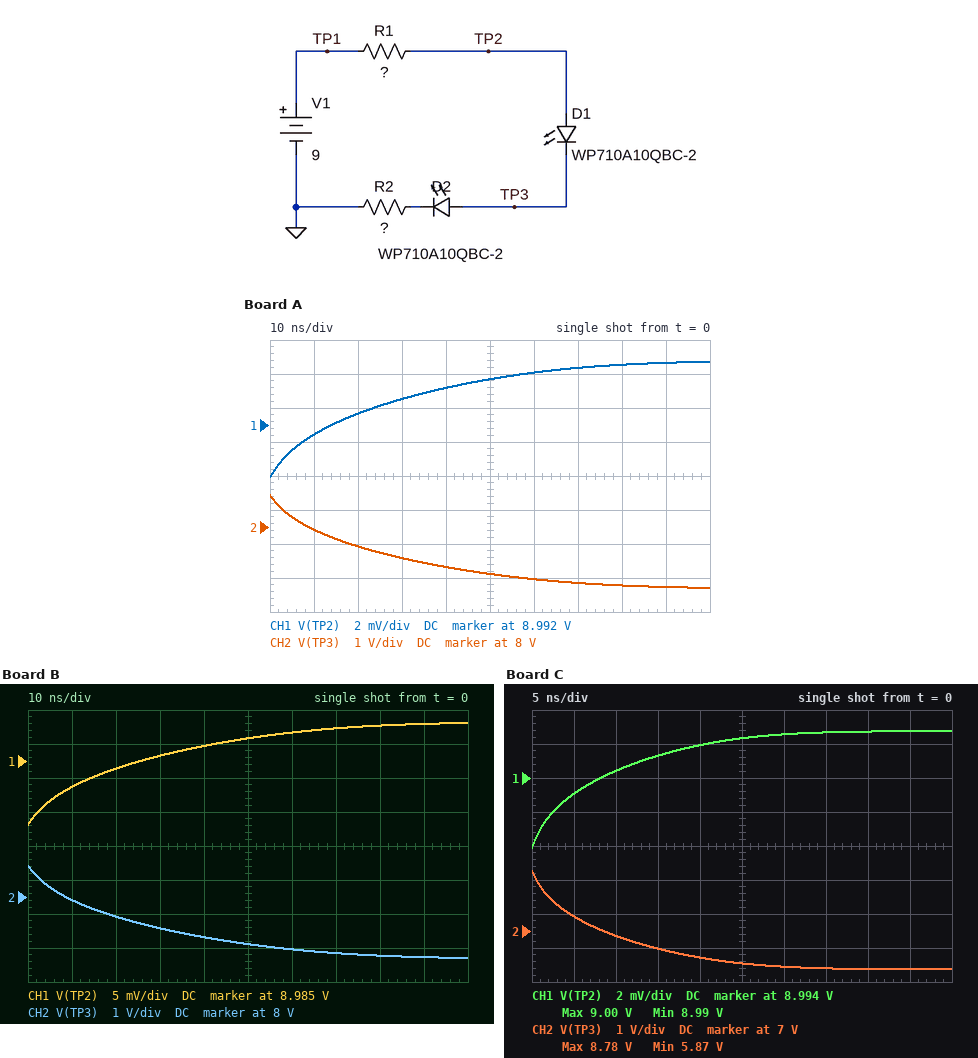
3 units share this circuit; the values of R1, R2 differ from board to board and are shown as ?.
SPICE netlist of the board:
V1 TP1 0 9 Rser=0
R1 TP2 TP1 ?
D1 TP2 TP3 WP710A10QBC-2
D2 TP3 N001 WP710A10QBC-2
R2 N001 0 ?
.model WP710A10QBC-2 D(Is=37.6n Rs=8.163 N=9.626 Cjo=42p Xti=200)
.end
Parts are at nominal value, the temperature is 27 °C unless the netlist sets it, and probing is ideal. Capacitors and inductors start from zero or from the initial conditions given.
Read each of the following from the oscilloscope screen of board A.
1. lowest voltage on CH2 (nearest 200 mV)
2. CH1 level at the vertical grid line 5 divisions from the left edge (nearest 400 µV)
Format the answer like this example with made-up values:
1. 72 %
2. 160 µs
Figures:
1. 6.2 V
2. 8.9948 V
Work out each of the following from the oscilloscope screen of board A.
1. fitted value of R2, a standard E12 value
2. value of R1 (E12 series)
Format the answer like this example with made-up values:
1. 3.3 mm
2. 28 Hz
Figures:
1. 1.2 kΩ
2. 1.5 Ω
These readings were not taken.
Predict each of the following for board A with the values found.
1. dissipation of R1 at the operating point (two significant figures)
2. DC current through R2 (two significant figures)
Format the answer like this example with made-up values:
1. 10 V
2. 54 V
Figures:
1. 12 µW
2. 2.8 mA
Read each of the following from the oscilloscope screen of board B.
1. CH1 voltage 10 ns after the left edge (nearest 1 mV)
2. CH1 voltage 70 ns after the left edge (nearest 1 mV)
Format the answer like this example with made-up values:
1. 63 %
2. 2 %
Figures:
1. 8.981 V
2. 8.990 V
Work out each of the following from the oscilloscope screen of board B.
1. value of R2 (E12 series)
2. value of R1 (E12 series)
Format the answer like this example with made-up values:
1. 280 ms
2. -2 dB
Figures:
1. 1.2 kΩ
2. 3.3 Ω
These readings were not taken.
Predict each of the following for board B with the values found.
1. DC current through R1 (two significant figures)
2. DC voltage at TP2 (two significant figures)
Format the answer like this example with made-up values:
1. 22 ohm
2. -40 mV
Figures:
1. 2.8 mA
2. 9.0 V
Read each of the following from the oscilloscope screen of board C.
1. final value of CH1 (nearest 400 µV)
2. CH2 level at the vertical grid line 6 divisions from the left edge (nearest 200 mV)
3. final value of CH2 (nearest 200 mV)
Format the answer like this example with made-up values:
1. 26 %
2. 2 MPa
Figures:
1. 8.9968 V
2. 6.0 V
3. 5.8 V
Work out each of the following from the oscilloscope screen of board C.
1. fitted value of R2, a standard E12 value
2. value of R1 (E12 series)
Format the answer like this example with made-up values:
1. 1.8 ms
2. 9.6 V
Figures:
1. 330 Ω
2. 0.39 Ω
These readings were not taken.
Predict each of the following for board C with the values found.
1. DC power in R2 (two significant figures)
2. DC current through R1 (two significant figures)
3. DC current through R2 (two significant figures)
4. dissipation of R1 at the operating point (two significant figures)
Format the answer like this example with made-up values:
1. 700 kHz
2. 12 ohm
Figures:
1. 23 mW
2. 8.3 mA
3. 8.3 mA
4. 27 µW
